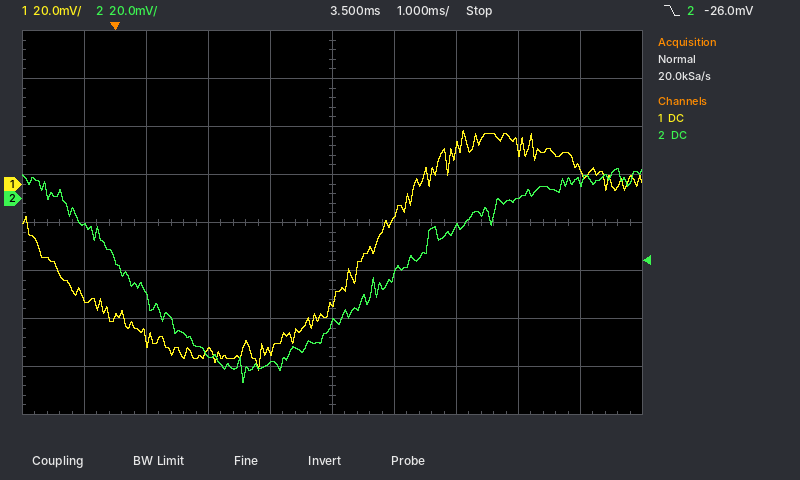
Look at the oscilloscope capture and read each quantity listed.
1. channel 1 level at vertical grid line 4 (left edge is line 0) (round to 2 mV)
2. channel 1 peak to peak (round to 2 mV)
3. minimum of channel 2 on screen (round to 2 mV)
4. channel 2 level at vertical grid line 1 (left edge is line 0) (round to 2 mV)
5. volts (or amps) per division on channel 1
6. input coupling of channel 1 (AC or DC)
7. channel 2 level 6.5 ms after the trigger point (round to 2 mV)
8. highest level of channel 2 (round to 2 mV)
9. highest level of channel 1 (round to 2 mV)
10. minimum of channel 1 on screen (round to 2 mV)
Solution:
-70 mV
100 mV
-76 mV
-12 mV
20 mV
DC
0 mV
12 mV
22 mV
-78 mV
